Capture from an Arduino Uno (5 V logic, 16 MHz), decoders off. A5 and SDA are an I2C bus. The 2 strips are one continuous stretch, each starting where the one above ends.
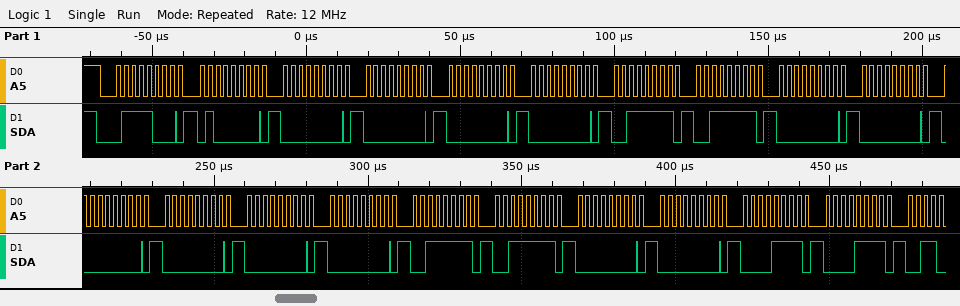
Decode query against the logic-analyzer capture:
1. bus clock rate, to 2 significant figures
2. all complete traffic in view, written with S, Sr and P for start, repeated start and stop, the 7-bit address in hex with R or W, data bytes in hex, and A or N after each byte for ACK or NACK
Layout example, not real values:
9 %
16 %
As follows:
400 kHz
S 3CW A 40 A 00 A 00 A 00 A 00 A 3F A 3F A 00 A 00 A 00 A 00 A 00 A 00 A 3F A 3F A 00 A 00 A 0F A 0F A
